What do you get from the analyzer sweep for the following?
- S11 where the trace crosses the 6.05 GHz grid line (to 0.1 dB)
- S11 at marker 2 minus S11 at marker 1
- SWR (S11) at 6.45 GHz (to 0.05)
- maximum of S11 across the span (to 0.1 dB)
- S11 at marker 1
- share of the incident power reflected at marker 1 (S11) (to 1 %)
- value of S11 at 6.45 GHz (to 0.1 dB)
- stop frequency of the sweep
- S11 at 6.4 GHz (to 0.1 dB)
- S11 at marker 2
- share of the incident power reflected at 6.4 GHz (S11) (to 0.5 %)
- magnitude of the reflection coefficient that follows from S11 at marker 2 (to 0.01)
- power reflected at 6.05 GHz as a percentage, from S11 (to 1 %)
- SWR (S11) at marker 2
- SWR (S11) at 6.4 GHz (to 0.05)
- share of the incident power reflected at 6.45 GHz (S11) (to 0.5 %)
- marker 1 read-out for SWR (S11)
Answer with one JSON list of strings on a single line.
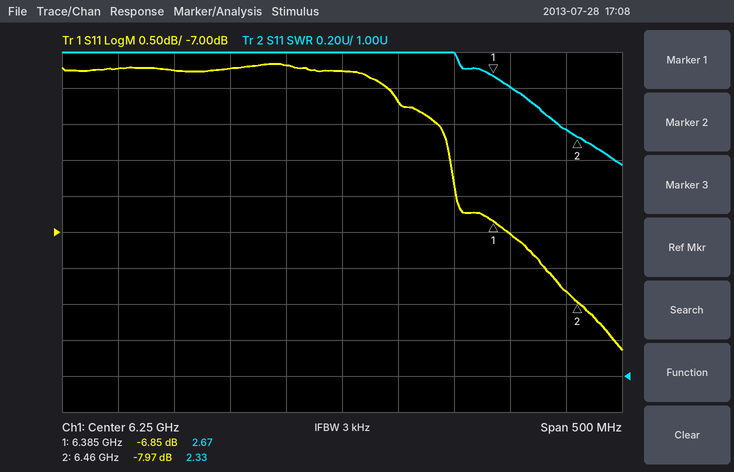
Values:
["-4.7 dB", "-1.12 dB", "2.35", "-4.7 dB", "-6.85 dB", "21 %", "-7.8 dB", "6.5 GHz", "-7.0 dB", "-7.97 dB", "20.0 %", "0.40", "34 %", "2.33", "2.60", "16.5 %", "2.67"]
